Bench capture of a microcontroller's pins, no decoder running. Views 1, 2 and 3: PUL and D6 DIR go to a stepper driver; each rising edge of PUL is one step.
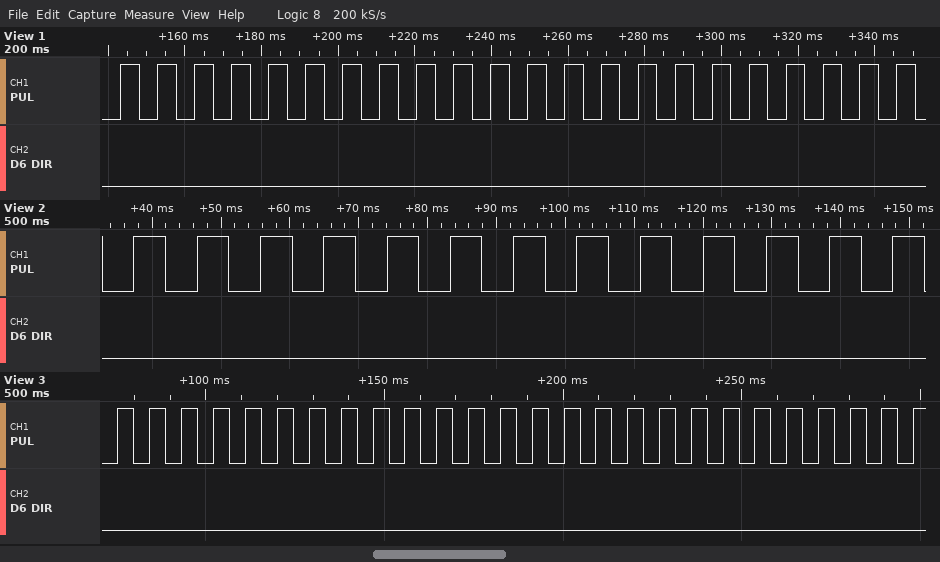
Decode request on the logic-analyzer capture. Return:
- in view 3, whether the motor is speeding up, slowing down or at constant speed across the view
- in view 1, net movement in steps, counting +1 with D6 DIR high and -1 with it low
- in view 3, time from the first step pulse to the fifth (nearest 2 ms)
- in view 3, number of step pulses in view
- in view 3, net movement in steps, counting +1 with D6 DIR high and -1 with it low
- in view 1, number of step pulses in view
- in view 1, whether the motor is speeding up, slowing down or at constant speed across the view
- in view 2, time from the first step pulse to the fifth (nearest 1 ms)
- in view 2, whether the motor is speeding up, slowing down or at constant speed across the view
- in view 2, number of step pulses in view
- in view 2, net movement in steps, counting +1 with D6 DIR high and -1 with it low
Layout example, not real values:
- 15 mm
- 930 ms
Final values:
- constant speed
- -22
- 36 ms
- 26
- -26
- 22
- constant speed
- 37 ms
- constant speed
- 13
- -13
